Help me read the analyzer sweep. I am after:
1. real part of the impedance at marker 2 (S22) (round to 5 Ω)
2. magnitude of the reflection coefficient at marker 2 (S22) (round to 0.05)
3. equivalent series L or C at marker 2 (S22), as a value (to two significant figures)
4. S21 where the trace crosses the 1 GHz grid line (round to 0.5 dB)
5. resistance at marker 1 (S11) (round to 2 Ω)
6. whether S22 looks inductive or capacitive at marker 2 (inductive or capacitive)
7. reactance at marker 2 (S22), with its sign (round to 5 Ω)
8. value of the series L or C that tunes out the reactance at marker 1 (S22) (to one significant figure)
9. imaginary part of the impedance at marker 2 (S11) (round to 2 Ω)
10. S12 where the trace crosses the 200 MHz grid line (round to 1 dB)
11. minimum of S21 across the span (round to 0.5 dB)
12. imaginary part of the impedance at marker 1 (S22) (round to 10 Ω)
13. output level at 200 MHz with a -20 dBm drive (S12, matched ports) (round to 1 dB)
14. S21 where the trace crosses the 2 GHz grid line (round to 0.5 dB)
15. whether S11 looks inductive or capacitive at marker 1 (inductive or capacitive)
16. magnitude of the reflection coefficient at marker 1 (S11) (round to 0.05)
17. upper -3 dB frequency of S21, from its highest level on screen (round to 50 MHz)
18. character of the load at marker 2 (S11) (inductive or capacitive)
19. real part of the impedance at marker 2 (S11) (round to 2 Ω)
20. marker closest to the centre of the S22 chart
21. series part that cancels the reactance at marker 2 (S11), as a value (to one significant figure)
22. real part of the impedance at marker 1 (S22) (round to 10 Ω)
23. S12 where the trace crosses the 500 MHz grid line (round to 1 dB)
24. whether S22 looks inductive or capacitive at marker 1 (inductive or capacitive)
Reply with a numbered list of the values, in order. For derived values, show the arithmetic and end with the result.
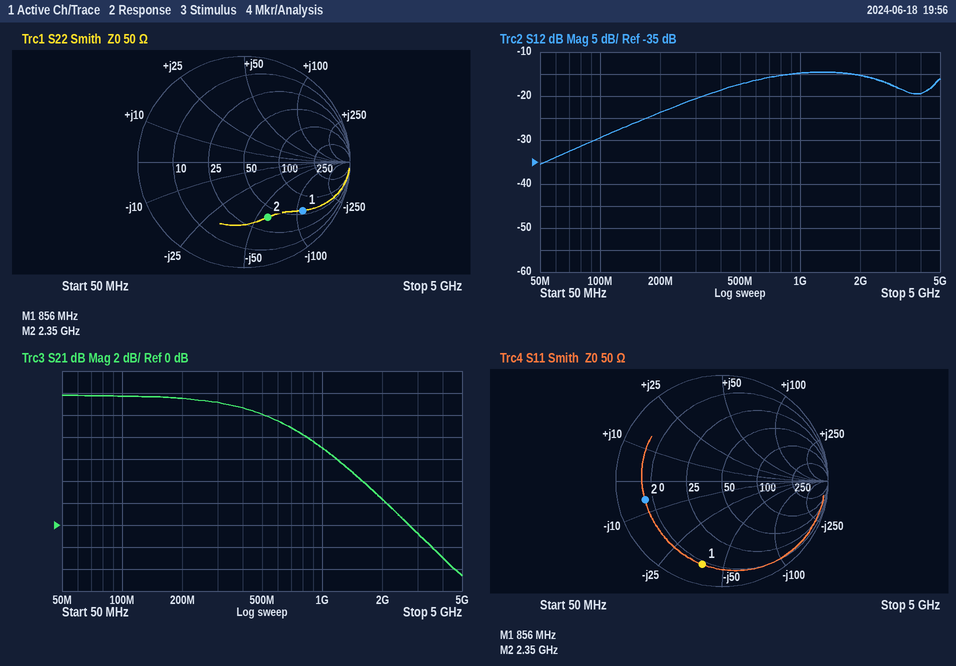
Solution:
1. 40 Ω
2. 0.55
3. C = 1/(2π × 2.35 GHz × 60 Ω) ≈ 1.1 pF
4. 7.0 dB
5. 8 Ω
6. capacitive
7. -60 Ω
8. L = 110 Ω/(2π × 856 MHz) ≈ 20 nH
9. -6 Ω
10. -24 dB
11. -4.5 dB
12. -110 Ω
13. -20 dBm + (-24 dB) = -44 dBm
14. 2.5 dB
15. capacitive
16. 0.80
17. 700 MHz
18. capacitive
19. 8 Ω
20. marker 2
21. L = 6 Ω/(2π × 2.35 GHz) ≈ 406 pH, so 400 pH to one significant figure
22. 60 Ω
23. -17 dB
24. capacitive
